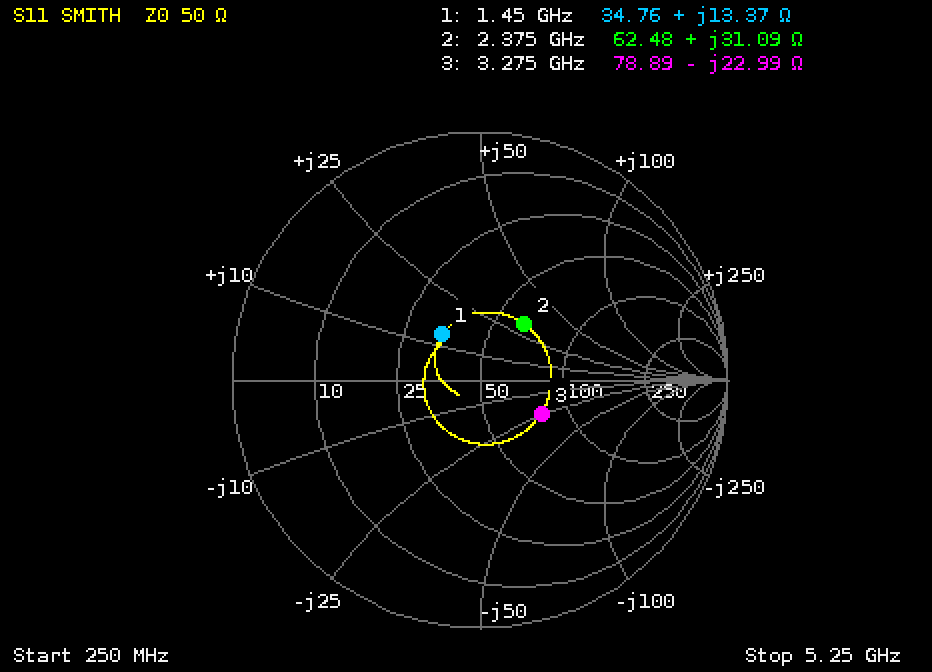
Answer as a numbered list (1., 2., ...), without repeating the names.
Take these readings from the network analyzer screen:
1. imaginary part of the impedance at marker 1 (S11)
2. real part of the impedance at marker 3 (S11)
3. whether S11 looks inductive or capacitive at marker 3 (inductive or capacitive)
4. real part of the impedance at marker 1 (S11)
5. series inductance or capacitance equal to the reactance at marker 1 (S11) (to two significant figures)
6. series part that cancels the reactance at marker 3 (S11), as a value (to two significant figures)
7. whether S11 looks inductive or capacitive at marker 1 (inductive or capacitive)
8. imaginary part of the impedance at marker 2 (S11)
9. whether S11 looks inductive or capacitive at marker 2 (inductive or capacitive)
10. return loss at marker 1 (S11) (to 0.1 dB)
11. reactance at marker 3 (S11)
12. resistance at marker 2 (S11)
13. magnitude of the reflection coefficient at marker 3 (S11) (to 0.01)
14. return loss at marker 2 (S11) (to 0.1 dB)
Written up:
1. +13.37 Ω
2. 78.89 Ω
3. capacitive
4. 34.76 Ω
5. 1.5 nH
6. 1.1 nH
7. inductive
8. +31.09 Ω
9. inductive
10. 12.5 dB
11. -22.99 Ω
12. 62.48 Ω
13. 0.28
14. 10.8 dB
